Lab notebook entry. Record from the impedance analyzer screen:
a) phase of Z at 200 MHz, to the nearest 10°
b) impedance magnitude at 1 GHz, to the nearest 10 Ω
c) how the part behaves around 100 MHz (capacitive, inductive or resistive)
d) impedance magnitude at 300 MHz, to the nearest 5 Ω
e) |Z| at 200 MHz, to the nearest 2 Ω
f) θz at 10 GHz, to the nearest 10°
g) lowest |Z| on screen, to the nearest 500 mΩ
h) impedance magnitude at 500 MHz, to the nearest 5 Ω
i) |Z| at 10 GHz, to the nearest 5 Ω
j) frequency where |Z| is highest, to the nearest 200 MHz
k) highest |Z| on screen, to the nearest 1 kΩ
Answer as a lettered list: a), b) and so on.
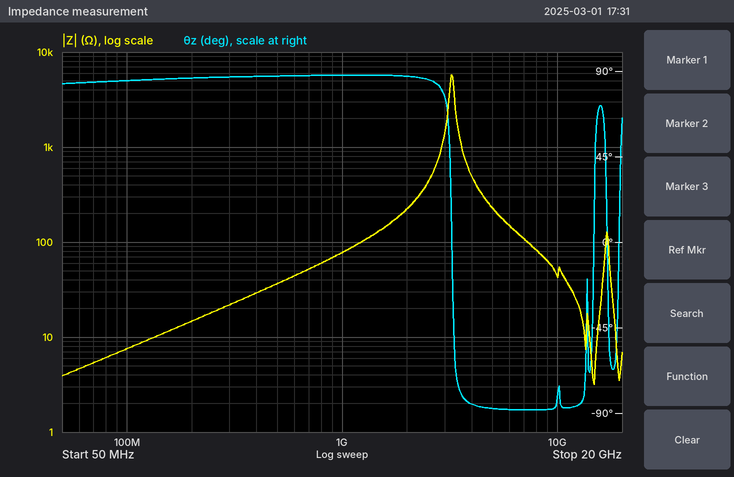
a) 90°
b) 80 Ω
c) inductive
d) 20 Ω
e) 14 Ω
f) -80°
g) 3.0 Ω
h) 35 Ω
i) 45 Ω
j) 3.2 GHz
k) 6 kΩ
